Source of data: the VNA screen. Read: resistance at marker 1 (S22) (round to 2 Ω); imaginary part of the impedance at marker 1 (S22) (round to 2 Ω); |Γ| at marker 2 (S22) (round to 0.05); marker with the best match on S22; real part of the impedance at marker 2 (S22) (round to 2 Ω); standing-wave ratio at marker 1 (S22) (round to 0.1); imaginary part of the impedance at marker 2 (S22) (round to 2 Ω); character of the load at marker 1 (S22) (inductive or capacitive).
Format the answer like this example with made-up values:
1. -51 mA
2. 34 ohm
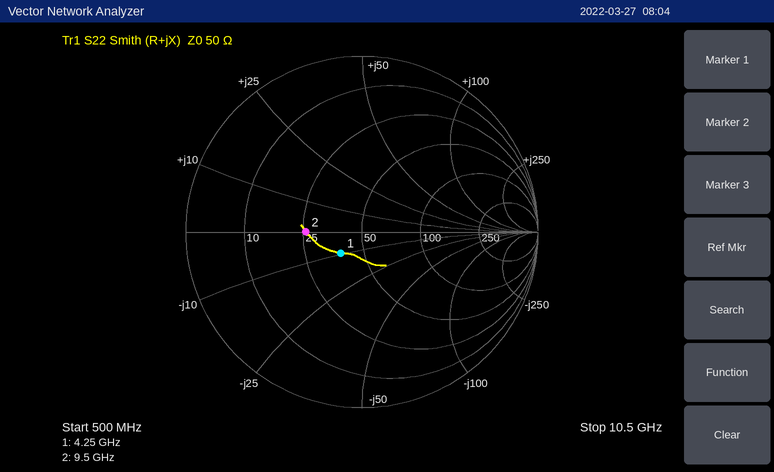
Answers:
1. 38 Ω
2. -10 Ω
3. 0.30
4. marker 1
5. 26 Ω
6. 1.4
7. 0 Ω
8. capacitive
